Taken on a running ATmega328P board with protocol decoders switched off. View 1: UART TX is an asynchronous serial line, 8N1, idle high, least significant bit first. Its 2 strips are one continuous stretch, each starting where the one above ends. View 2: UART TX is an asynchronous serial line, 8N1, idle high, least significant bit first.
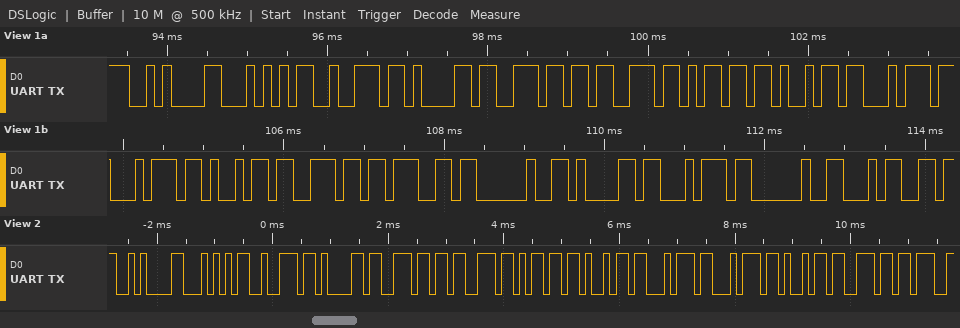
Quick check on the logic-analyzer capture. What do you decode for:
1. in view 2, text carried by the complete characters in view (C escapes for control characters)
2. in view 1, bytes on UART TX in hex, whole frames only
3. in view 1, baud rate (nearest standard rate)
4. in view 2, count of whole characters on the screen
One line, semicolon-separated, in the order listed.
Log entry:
"\nTransmittin"; 0A 54 72 61 6E 73 6D 69 74 74 69 6E 67 20 61 74 20 34; 9600 baud; 12
